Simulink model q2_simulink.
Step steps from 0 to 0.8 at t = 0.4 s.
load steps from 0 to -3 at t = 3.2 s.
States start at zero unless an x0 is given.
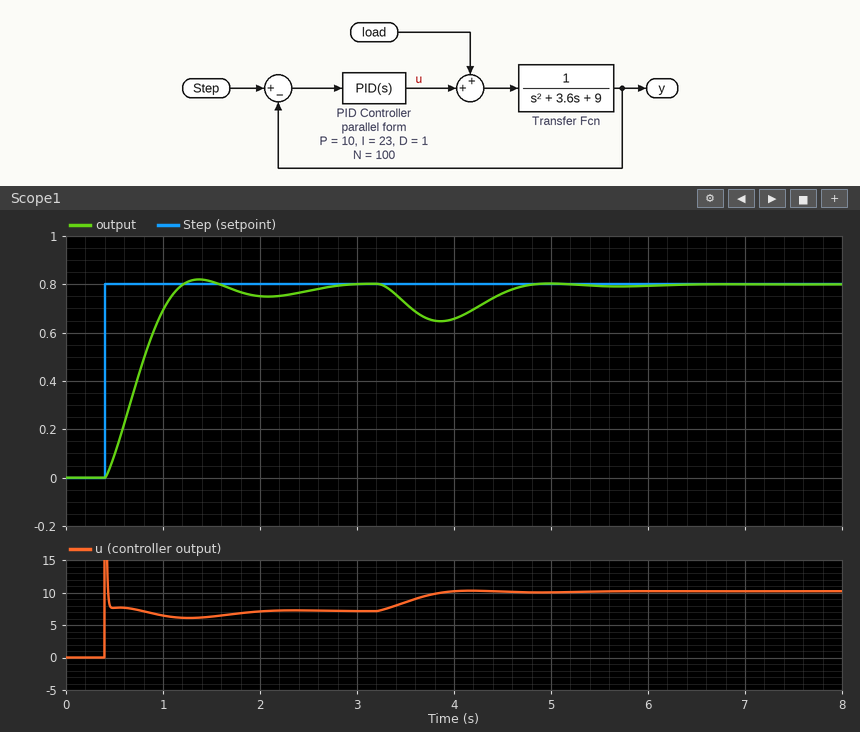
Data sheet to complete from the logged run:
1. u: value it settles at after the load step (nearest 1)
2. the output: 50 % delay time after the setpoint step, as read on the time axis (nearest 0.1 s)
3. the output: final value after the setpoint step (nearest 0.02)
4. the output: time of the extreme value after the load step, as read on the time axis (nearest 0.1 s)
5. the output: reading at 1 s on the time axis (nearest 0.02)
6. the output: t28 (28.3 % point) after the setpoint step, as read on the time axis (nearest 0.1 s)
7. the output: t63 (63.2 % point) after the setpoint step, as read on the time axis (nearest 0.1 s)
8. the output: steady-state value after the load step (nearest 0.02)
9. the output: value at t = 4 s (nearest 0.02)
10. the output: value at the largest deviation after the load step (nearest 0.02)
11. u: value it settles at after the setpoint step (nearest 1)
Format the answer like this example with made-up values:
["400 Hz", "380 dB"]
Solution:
["10", "0.7 s", "0.80", "3.9 s", "0.70", "0.6 s", "0.8 s", "0.80", "0.66", "0.64", "7"]
